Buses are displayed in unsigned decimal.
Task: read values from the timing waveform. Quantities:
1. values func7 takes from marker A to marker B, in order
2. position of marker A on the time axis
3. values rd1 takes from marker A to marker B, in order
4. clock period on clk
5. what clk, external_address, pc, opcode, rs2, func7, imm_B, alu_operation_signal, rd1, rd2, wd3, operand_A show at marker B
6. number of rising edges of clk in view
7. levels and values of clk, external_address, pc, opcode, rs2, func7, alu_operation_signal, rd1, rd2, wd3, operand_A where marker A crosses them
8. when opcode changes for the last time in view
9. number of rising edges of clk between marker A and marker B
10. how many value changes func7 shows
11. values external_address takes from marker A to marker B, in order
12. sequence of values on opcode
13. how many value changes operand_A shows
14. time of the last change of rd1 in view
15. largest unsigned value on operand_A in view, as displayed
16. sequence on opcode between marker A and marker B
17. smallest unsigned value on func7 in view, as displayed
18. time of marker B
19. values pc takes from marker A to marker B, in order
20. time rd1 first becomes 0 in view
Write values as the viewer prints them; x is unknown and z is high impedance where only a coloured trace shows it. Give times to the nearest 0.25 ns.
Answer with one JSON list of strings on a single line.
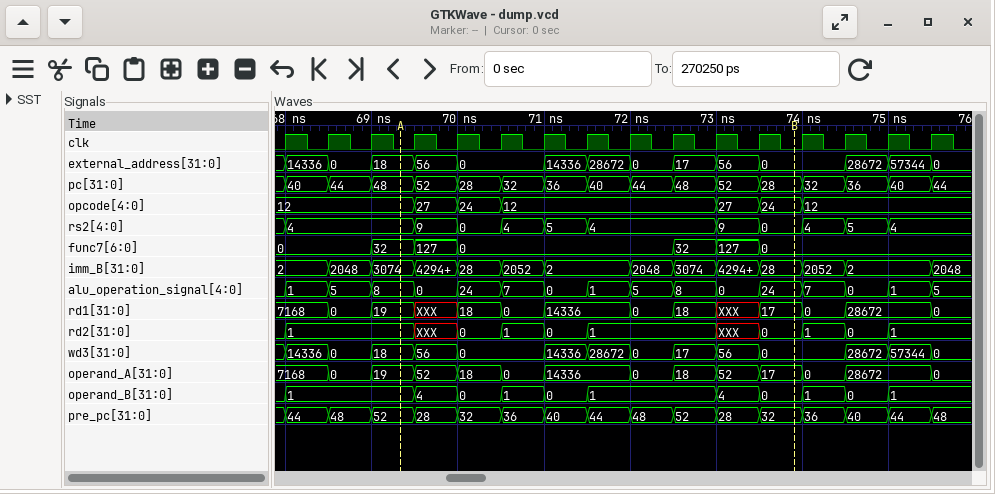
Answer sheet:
["32, 127, 0, 32, 127, 0", "69.25 ns", "19, XXX, 18, 0, 14336, 0, 18, XXX, 17", "0.5 ns", "clk=0, external_address=0, pc=28, opcode=24, rs2=0, func7=0, imm_B=28, alu_operation_signal=24, rd1=17, rd2=0, wd3=0, operand_A=17", "16", "clk=0, external_address=18, pc=48, opcode=12, rs2=4, func7=32, alu_operation_signal=8, rd1=19, rd2=1, wd3=18, operand_A=19", "74 ns", "9", "6", "18, 56, 0, 14336, 28672, 0, 17, 56, 0", "12, 27, 24, 12, 27, 24, 12", "13", "75.5 ns", "28672", "12, 27, 24, 12, 27, 24", "0", "74 ns", "48, 52, 28, 32, 36, 40, 44, 48, 52, 28", "68.5 ns"]
